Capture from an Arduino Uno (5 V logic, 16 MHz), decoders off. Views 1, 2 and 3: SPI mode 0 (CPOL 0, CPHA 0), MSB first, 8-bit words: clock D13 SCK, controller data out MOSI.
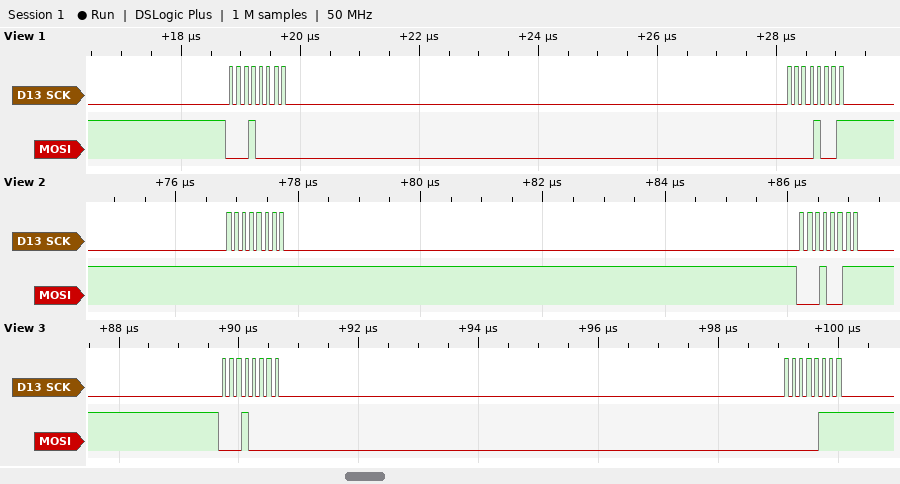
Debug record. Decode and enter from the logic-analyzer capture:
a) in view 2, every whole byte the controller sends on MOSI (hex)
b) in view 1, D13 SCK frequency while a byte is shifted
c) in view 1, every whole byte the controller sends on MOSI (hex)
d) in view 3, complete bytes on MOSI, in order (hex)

FF 13
8 MHz
10 09
10 07
